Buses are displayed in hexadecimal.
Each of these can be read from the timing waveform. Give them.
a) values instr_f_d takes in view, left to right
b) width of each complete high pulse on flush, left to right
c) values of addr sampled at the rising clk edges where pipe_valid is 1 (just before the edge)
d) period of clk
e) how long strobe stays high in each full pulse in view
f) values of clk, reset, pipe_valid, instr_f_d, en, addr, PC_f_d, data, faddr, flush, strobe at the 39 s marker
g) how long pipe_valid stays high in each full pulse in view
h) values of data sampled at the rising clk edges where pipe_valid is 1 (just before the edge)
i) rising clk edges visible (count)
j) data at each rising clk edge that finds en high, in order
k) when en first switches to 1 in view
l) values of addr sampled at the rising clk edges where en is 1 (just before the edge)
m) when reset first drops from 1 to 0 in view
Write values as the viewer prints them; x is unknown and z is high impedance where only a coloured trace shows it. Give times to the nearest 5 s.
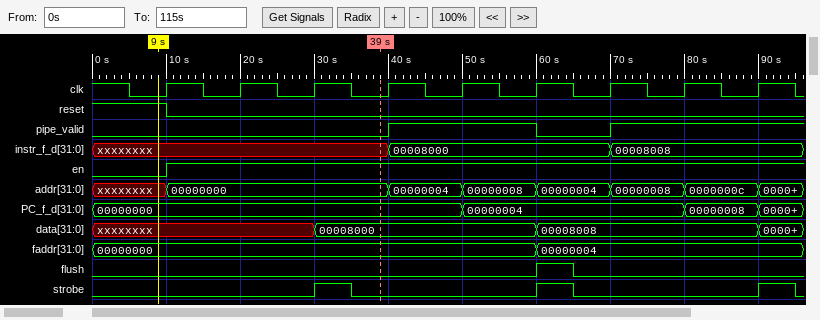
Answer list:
xxxxxxxx, 00008000, 00008008
5 s
00000004, 00000008, 00000008, 0000000c
10 s
5 s, 5 s, 5 s
clk=0, reset=0, pipe_valid=0, instr_f_d=xxxxxxxx, en=1, addr=00000000, PC_f_d=00000000, data=00008000, faddr=00000000, flush=0, strobe=0
20 s
00008000, 00008000, 00008008, 00008008
9
xxxxxxxx, xxxxxxxx, 00008000, 00008000, 00008000, 00008008, 00008008, 00008008
10 s
00000000, 00000000, 00000000, 00000004, 00000008, 00000004, 00000008, 0000000c
10 s
